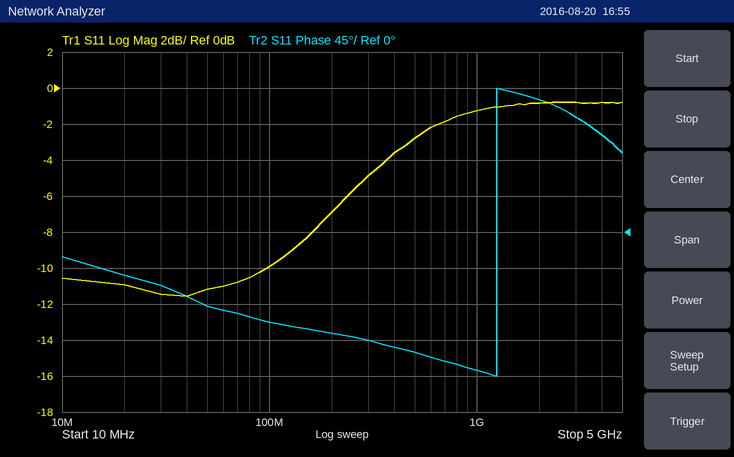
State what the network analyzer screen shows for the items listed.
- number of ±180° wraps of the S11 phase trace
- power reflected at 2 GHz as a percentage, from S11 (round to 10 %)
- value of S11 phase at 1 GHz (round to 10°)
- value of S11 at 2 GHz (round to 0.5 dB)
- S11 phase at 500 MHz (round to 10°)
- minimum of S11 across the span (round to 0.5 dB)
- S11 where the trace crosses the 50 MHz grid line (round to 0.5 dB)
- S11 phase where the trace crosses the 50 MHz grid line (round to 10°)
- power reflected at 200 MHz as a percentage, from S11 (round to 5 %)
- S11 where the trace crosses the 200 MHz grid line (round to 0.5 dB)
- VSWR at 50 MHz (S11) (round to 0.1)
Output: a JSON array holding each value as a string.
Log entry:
["1", "80 %", "-170°", "-1.0 dB", "-150°", "-11.5 dB", "-11.0 dB", "-90°", "20 %", "-7.0 dB", "1.8"]
